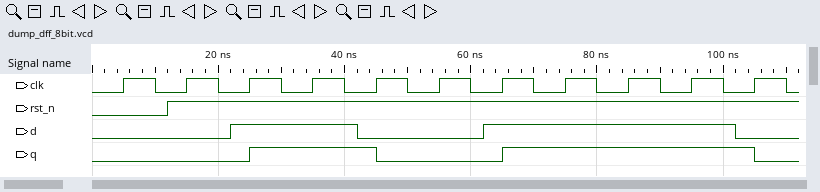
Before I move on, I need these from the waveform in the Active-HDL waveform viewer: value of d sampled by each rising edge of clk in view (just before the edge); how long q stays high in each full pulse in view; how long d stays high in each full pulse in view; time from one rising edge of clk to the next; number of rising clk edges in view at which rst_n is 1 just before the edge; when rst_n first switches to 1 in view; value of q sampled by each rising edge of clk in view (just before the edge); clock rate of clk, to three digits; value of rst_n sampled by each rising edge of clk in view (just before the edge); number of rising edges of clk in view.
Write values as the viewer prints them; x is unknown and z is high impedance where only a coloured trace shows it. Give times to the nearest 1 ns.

0 0 1 1 0 0 1 1 1 1 0
20 ns, 40 ns
20 ns, 40 ns
10 ns
10
12 ns
0 0 0 1 1 0 0 1 1 1 1
100 MHz
0 1 1 1 1 1 1 1 1 1 1
11
